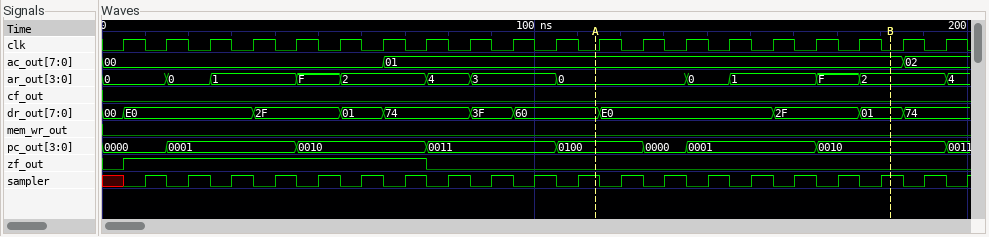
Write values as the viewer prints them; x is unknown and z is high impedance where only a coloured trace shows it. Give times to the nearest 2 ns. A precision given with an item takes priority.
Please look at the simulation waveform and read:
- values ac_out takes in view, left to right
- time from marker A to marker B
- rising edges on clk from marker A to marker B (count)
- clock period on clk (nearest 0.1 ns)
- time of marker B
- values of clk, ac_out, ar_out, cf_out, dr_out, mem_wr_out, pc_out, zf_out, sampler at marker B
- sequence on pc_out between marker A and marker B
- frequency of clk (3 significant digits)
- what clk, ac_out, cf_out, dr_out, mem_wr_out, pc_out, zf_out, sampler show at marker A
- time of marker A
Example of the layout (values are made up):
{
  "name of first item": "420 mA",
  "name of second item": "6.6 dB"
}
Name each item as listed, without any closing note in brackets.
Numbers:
{
  "values ac_out takes in view, left to right": "00, 01, 02",
  "time from marker A to marker B": "68 ns",
  "rising edges on clk from marker A to marker B": "7",
  "clock period on clk": "10 ns",
  "time of marker B": "182 ns",
  "values of clk, ac_out, ar_out, cf_out, dr_out, mem_wr_out, pc_out, zf_out, sampler at marker B": "clk=0, ac_out=01, ar_out=2, cf_out=0, dr_out=01, mem_wr_out=0, pc_out=0010, zf_out=0, sampler=1",
  "sequence on pc_out between marker A and marker B": "0100, 0000, 0001, 0010",
  "frequency of clk": "100 MHz",
  "what clk, ac_out, cf_out, dr_out, mem_wr_out, pc_out, zf_out, sampler show at marker A": "clk=0, ac_out=01, cf_out=0, dr_out=60, mem_wr_out=0, pc_out=0100, zf_out=0, sampler=1",
  "time of marker A": "114 ns"
}
